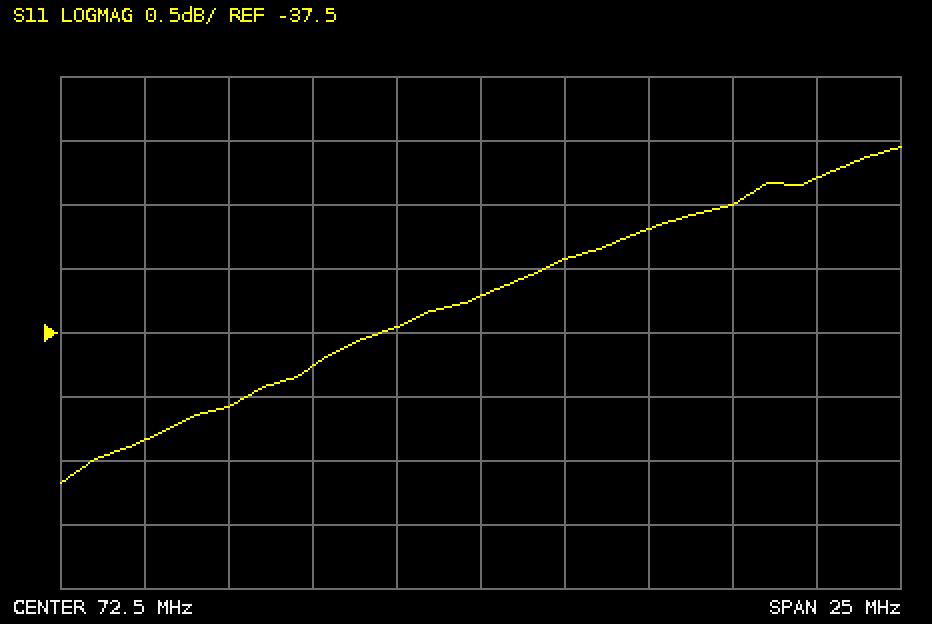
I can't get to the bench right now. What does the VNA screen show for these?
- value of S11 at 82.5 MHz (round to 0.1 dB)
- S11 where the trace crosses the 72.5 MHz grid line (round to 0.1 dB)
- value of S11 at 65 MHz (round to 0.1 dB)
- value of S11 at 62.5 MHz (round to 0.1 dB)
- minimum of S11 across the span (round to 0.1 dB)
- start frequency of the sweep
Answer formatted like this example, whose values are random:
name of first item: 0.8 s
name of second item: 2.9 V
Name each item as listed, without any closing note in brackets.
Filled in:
value of S11 at 82.5 MHz: -36.3 dB
S11 where the trace crosses the 72.5 MHz grid line: -37.2 dB
value of S11 at 65 MHz: -38.1 dB
value of S11 at 62.5 MHz: -38.3 dB
minimum of S11 across the span: -38.7 dB
start frequency of the sweep: 60 MHz
